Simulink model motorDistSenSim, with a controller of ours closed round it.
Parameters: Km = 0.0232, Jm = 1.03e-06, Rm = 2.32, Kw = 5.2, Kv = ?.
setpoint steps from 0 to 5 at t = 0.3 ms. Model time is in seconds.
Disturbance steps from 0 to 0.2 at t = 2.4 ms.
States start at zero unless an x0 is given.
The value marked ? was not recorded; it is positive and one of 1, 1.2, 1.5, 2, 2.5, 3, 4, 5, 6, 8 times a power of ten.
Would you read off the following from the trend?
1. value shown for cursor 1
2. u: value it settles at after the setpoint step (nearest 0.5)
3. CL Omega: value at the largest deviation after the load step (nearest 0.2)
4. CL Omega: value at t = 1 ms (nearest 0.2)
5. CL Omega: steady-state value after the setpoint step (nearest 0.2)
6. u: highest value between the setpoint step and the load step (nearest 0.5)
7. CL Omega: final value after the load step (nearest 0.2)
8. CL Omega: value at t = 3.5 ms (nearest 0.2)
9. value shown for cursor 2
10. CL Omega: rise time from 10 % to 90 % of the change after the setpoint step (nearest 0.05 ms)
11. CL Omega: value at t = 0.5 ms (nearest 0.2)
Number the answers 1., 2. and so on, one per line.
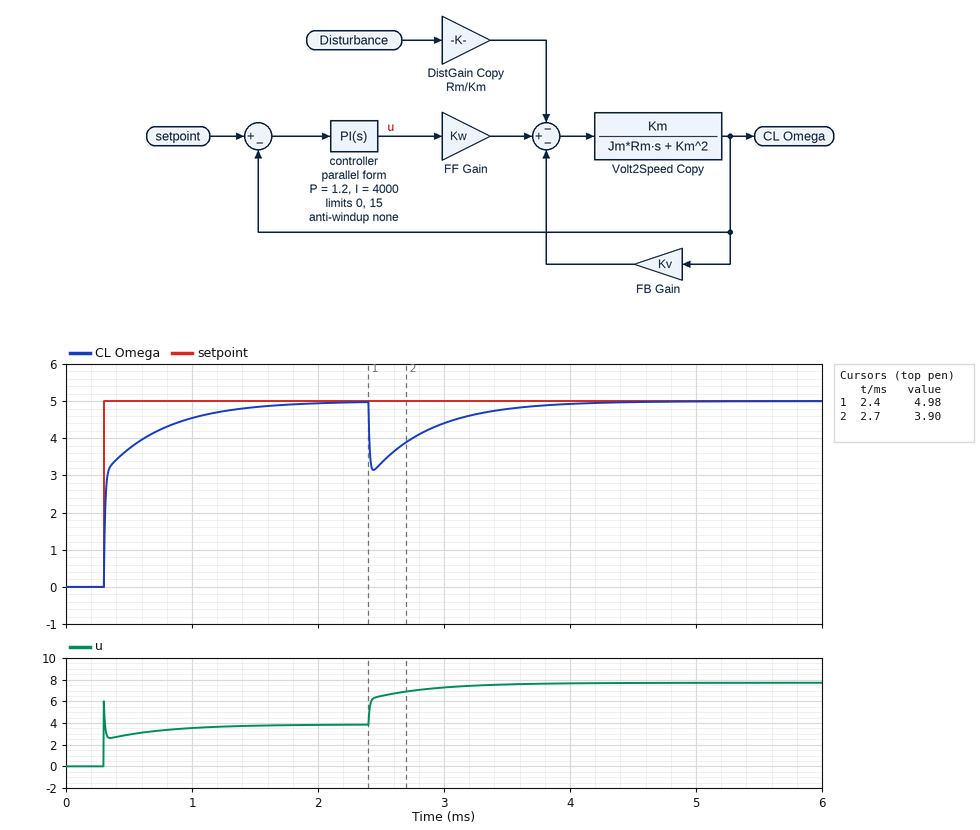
1. 4.98
2. 4.0
3. 3.2
4. 4.6
5. 5.0
6. 6.0
7. 5.0
8. 4.8
9. 3.90
10. 0.65 ms
11. 3.8
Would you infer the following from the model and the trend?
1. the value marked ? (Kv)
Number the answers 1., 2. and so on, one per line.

1. 4
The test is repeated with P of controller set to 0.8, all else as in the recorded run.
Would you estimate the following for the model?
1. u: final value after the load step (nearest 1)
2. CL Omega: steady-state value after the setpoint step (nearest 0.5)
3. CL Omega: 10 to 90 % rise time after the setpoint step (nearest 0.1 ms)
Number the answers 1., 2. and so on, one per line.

1. 8
2. 5.0
3. 0.6 ms
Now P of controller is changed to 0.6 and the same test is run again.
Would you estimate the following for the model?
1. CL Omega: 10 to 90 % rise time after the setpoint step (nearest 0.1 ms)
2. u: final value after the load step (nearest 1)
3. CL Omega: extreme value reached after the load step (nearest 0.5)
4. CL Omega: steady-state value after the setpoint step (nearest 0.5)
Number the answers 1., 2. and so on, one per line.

1. 0.6 ms
2. 8
3. 2.5
4. 5.0
